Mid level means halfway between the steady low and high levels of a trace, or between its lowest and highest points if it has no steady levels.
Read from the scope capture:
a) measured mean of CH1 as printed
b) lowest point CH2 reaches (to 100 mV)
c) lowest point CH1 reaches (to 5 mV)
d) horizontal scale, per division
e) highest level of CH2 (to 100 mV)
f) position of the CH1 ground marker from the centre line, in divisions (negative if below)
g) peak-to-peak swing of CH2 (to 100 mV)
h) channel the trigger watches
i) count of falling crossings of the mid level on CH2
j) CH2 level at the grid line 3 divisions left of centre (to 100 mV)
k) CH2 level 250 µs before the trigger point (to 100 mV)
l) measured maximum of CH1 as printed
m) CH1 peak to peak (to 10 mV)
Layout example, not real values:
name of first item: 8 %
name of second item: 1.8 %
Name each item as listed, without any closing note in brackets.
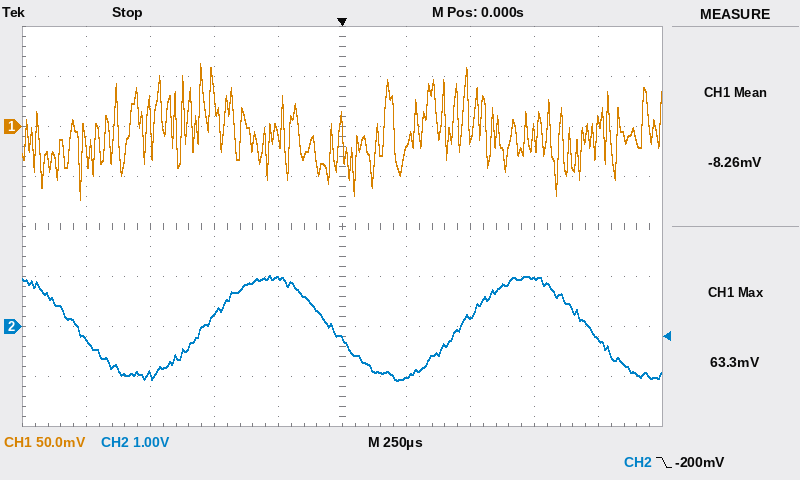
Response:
measured mean of CH1 as printed: -8.26 mV
lowest point CH2 reaches: -1.1 V
lowest point CH1 reaches: -75 mV
horizontal scale, per division: 250 µs
highest level of CH2: 1.0 V
position of the CH1 ground marker from the centre line, in divisions: +2.0 div
peak-to-peak swing of CH2: 2.1 V
channel the trigger watches: CH2
count of falling crossings of the mid level on CH2: 3
CH2 level at the grid line 3 divisions left of centre: -1.0 V
CH2 level 250 µs before the trigger point: 1.0 V
measured maximum of CH1 as printed: 63.3 mV
CH1 peak to peak: 140 mV
